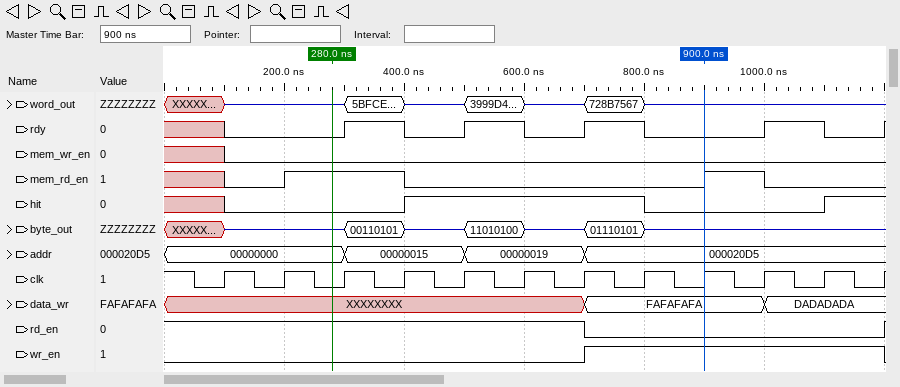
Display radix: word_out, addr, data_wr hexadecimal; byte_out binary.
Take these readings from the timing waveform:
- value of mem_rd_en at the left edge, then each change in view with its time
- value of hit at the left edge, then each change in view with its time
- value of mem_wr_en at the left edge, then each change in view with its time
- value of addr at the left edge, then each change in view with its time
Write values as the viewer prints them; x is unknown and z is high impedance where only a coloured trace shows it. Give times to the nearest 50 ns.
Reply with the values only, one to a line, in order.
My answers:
x, 0 at 100 ns, 1 at 200 ns, 0 at 400 ns, 1 at 900 ns, 0 at 1000 ns
x, 0 at 100 ns, 1 at 400 ns, 0 at 800 ns, 1 at 1100 ns
x, 0 at 100 ns
00000000, 00000015 at 300 ns, 00000019 at 500 ns, 000020D5 at 700 ns
